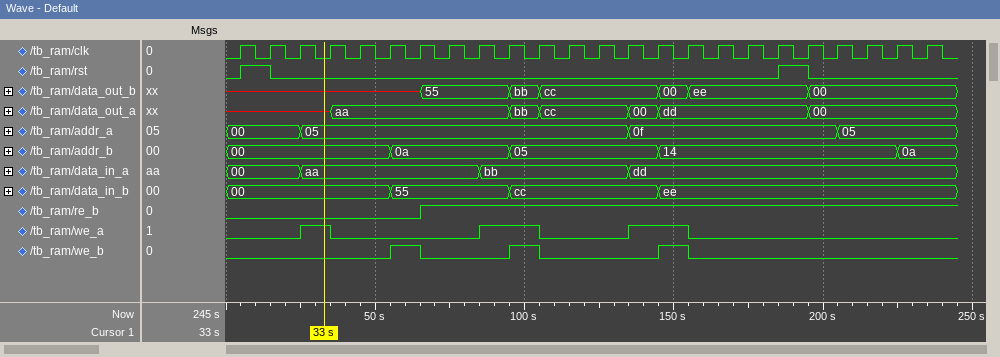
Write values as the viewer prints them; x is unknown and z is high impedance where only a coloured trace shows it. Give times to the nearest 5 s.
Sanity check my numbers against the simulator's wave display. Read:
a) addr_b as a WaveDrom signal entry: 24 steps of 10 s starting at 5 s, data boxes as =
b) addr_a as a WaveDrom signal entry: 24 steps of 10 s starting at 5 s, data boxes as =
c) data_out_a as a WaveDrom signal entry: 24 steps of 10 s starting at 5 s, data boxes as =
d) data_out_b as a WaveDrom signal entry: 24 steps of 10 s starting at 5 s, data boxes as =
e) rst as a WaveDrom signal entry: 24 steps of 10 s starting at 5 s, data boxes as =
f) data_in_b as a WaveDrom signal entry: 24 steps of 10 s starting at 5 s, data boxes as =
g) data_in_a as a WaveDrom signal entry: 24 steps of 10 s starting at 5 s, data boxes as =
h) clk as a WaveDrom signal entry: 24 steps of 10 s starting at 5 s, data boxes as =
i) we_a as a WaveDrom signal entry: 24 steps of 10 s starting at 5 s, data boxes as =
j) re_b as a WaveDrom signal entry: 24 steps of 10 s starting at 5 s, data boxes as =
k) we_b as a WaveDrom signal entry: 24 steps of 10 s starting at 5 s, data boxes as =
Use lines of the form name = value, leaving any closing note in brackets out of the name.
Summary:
addr_b as a WaveDrom signal entry: 24 steps of 10 s starting at 5 s, data boxes as = = {name: 'addr_b', wave: '=....=...=....=.......=.', data: '00 0a 05 14 0a'}
addr_a as a WaveDrom signal entry: 24 steps of 10 s starting at 5 s, data boxes as = = {name: 'addr_a', wave: '=.=..........=......=...', data: '00 05 0f 05'}
data_out_a as a WaveDrom signal entry: 24 steps of 10 s starting at 5 s, data boxes as = = {name: 'data_out_a', wave: 'x..=.....==..==....=....', data: 'aa bb cc 00 dd 00'}
data_out_b as a WaveDrom signal entry: 24 steps of 10 s starting at 5 s, data boxes as = = {name: 'data_out_b', wave: 'x.....=..==...==...=....', data: '55 bb cc 00 ee 00'}
rst as a WaveDrom signal entry: 24 steps of 10 s starting at 5 s, data boxes as = = {name: 'rst', wave: '10................10....'}
data_in_b as a WaveDrom signal entry: 24 steps of 10 s starting at 5 s, data boxes as = = {name: 'data_in_b', wave: '=....=...=....=.........', data: '00 55 cc ee'}
data_in_a as a WaveDrom signal entry: 24 steps of 10 s starting at 5 s, data boxes as = = {name: 'data_in_a', wave: '=.=.....=....=..........', data: '00 aa bb dd'}
clk as a WaveDrom signal entry: 24 steps of 10 s starting at 5 s, data boxes as = = {name: 'clk', wave: 'p.......................'}
we_a as a WaveDrom signal entry: 24 steps of 10 s starting at 5 s, data boxes as = = {name: 'we_a', wave: '0.10....1.0..1.0........'}
re_b as a WaveDrom signal entry: 24 steps of 10 s starting at 5 s, data boxes as = = {name: 're_b', wave: '0.....1.................'}
we_b as a WaveDrom signal entry: 24 steps of 10 s starting at 5 s, data boxes as = = {name: 'we_b', wave: '0....10..10...10........'}
